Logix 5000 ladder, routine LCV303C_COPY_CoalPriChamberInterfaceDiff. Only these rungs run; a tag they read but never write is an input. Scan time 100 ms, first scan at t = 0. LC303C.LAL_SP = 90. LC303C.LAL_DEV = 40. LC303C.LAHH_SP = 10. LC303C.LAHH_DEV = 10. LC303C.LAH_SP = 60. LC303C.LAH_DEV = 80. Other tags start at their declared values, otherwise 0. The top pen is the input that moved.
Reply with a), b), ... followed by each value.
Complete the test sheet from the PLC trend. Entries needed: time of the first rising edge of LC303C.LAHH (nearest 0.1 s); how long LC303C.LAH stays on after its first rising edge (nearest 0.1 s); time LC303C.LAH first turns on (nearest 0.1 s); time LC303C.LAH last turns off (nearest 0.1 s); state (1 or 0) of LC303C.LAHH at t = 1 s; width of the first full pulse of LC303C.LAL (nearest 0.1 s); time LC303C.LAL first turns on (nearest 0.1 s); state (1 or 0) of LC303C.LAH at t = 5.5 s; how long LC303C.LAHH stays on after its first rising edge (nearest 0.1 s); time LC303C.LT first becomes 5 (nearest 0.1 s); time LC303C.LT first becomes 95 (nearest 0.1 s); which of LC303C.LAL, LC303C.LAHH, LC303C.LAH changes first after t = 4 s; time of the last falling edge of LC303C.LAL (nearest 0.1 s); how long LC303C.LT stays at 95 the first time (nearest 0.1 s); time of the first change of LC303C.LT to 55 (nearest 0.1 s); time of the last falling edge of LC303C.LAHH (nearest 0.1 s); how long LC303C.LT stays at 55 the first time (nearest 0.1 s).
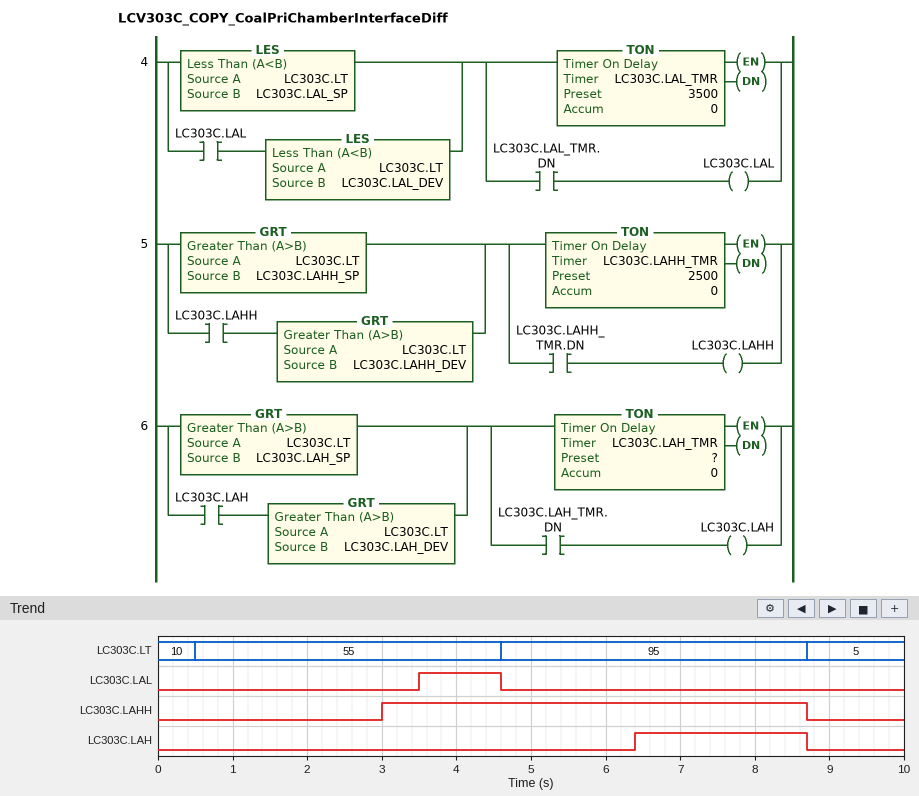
a) 3.0 s
b) 2.3 s
c) 6.4 s
d) 8.7 s
e) 0
f) 1.1 s
g) 3.5 s
h) 0
i) 5.7 s
j) 8.7 s
k) 4.6 s
l) LC303C.LAL
m) 4.6 s
n) 4.1 s
o) 0.5 s
p) 8.7 s
q) 4.1 s
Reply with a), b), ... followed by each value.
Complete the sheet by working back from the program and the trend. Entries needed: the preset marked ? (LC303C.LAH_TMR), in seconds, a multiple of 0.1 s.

a) 1.8 s
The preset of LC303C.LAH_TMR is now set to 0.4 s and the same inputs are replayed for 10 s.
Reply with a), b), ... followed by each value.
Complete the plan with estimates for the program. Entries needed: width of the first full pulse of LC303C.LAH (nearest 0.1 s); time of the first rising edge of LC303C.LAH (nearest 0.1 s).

a) 3.7 s
b) 5.0 s
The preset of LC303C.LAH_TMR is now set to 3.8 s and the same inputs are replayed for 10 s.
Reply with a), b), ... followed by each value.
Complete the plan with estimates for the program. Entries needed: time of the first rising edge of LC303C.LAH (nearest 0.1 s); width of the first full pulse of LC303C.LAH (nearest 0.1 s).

a) 8.4 s
b) 0.3 s
